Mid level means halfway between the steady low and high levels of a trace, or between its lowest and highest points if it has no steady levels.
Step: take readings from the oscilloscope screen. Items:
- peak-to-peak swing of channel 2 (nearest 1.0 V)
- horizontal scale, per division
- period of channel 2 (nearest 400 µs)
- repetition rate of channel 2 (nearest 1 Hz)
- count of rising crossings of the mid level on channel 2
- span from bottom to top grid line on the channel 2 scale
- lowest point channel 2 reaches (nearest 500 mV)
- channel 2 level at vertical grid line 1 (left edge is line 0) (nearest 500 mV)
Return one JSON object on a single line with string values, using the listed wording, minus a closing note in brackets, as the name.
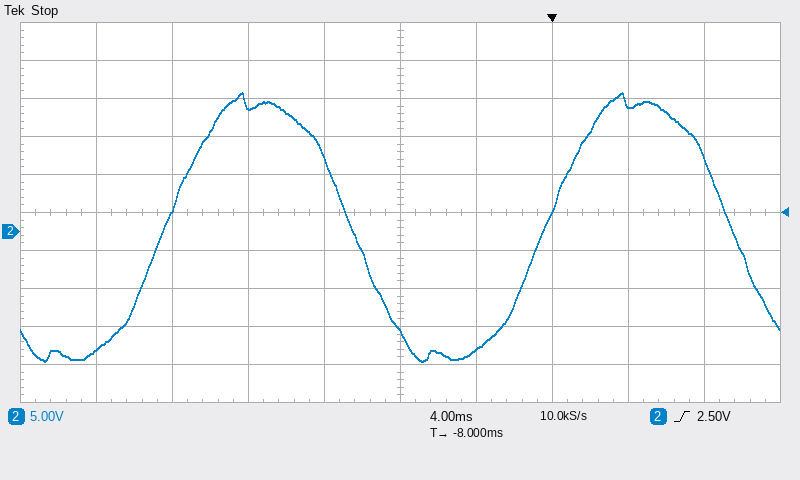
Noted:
{"peak-to-peak swing of channel 2": "35.0 V", "horizontal scale, per division": "4 ms", "period of channel 2": "20.0 ms", "repetition rate of channel 2": "50 Hz", "count of rising crossings of the mid level on channel 2": "2", "span from bottom to top grid line on the channel 2 scale": "50 V", "lowest point channel 2 reaches": "-17.0 V", "channel 2 level at vertical grid line 1 (left edge is line 0)": "-15.5 V"}
